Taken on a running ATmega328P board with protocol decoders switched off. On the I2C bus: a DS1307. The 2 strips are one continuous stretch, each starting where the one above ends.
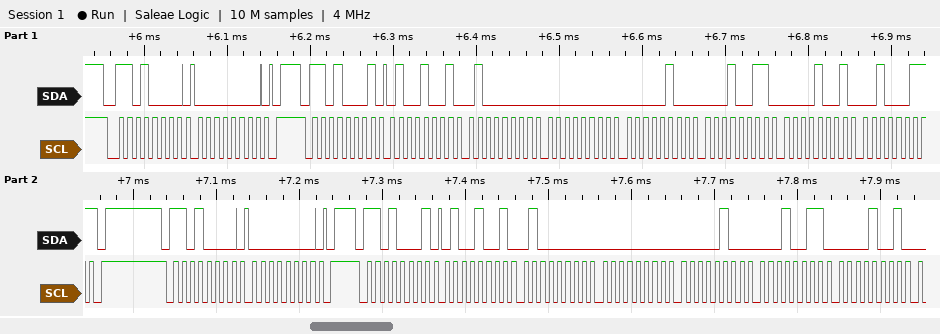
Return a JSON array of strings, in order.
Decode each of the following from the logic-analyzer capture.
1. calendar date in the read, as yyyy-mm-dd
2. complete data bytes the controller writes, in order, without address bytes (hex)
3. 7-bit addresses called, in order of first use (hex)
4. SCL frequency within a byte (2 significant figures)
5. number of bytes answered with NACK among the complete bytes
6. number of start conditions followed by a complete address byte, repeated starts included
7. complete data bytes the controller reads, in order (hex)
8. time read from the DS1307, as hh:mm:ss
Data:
["2023-09-13", "00 00", "0x68", "100 kHz", "1", "4", "49 40 00 04 13 09 23 49 40 00 04 13 09", "00:40:49"]
